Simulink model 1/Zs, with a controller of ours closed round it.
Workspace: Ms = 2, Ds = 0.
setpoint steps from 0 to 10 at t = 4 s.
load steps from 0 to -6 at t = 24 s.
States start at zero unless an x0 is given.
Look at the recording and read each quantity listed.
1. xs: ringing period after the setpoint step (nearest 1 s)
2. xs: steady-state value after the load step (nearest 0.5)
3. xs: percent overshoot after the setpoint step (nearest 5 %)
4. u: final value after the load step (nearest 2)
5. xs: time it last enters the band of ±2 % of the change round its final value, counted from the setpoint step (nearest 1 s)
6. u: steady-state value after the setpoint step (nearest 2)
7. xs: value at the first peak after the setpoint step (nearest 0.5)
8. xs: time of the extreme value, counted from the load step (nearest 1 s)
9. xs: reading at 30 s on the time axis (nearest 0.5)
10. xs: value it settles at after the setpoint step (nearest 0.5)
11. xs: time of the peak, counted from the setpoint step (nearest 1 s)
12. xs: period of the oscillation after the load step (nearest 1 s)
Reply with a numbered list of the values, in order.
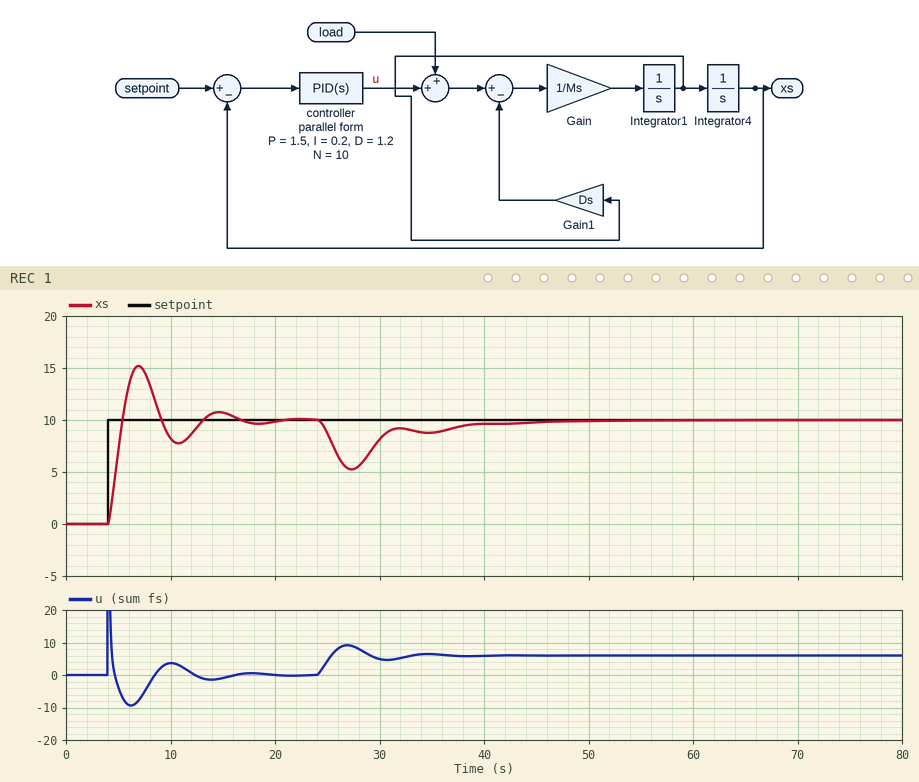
1. 8 s
2. 10.0
3. 50 %
4. 6
5. 16 s
6. 0
7. 15.0
8. 3 s
9. 8.0
10. 10.0
11. 3 s
12. 7 s
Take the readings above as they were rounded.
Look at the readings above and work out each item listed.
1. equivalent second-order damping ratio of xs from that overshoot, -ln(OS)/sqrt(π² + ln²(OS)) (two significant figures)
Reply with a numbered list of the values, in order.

1. 0.22
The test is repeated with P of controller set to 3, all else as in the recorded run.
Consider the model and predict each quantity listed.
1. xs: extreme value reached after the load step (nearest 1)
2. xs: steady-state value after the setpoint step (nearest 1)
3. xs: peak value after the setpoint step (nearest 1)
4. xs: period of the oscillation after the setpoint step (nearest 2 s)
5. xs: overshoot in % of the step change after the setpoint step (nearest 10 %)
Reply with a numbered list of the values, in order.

1. 7
2. 10
3. 16
4. 6 s
5. 60 %
